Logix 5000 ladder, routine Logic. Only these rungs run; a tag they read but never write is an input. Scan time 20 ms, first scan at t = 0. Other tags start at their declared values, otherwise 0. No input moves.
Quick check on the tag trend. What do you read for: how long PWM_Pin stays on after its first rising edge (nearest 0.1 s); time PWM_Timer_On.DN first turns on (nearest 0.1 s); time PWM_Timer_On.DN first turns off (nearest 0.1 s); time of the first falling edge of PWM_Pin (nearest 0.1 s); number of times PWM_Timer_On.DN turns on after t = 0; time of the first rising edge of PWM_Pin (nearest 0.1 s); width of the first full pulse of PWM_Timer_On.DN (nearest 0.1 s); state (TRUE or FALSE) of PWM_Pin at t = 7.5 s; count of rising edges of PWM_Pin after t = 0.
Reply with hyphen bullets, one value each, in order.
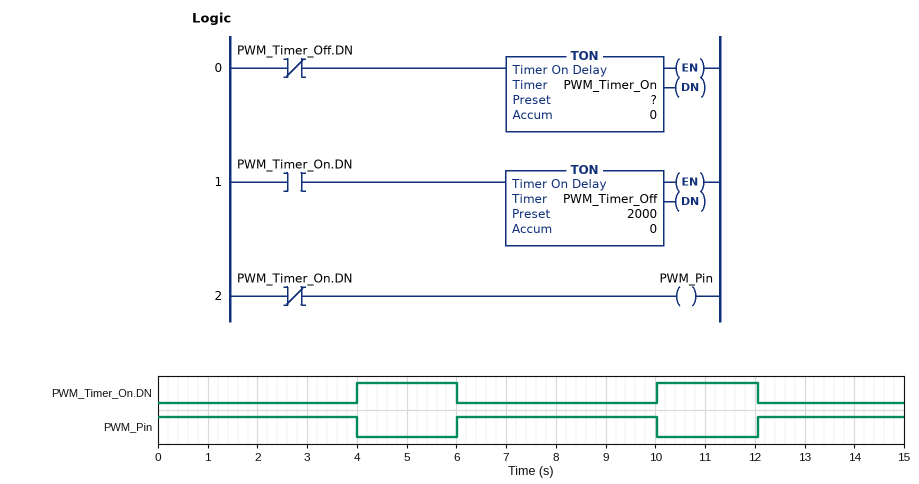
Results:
- 4.0 s
- 4.0 s
- 6.0 s
- 4.0 s
- 2
- 6.0 s
- 2.0 s
- TRUE
- 2
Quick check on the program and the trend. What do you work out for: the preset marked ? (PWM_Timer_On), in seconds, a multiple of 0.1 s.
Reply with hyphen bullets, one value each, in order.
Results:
- 4.0 s
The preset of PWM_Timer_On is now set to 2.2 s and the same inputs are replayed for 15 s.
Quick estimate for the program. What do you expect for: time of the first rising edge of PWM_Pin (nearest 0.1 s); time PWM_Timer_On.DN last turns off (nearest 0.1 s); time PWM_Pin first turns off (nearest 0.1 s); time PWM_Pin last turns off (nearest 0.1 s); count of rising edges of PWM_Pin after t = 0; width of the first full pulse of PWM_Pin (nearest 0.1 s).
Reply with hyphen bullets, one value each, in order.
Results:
- 4.2 s
- 12.7 s
- 2.2 s
- 14.9 s
- 3
- 2.2 s
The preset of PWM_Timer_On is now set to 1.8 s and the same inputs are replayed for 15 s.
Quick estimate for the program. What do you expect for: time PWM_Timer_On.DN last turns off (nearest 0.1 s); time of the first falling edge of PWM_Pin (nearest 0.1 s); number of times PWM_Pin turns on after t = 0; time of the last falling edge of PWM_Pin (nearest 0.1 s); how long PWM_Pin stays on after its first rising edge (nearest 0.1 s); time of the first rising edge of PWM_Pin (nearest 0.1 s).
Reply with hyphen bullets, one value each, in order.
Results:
- 11.5 s
- 1.8 s
- 3
- 13.3 s
- 1.8 s
- 3.8 s
